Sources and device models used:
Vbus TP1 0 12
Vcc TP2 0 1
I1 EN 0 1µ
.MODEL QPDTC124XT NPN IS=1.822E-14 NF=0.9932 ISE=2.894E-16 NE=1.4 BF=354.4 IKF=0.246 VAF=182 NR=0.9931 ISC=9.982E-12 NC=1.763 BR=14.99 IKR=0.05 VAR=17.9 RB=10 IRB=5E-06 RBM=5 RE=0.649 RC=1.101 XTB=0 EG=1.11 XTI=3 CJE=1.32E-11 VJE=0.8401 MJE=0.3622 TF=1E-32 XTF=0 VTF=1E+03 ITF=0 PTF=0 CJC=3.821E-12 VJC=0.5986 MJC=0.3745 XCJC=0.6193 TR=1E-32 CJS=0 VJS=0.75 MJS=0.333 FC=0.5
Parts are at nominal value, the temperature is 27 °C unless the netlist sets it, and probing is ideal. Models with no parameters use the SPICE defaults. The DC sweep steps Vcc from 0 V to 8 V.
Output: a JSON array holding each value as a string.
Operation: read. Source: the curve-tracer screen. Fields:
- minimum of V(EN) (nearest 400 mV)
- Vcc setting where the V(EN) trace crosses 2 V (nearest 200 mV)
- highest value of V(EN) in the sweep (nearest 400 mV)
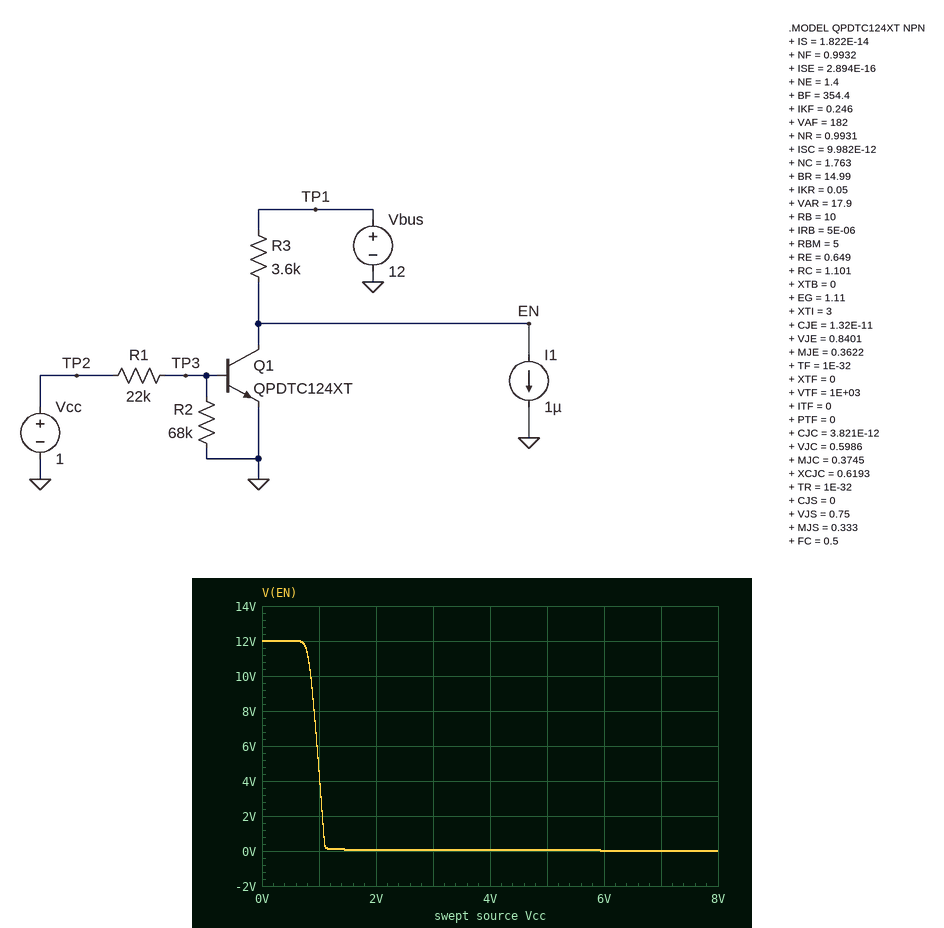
["0 V", "1.0 V", "12.0 V"]
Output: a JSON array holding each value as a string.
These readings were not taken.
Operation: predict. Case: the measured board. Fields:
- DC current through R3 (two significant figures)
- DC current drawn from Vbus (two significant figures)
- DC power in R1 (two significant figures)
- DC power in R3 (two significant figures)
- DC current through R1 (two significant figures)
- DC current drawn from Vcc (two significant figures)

["2.1 mA", "2.1 mA", "5.4 µW", "15 mW", "16 µA", "16 µA"]
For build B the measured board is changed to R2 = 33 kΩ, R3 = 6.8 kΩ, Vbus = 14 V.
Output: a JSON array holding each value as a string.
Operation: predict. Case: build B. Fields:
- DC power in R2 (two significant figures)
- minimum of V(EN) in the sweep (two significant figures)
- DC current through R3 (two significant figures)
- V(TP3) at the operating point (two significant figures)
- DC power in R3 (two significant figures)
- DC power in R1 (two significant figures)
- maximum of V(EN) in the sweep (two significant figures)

["11 µW", "17 mV", "200 µA", "590 mV", "270 µW", "7.5 µW", "14 V"]
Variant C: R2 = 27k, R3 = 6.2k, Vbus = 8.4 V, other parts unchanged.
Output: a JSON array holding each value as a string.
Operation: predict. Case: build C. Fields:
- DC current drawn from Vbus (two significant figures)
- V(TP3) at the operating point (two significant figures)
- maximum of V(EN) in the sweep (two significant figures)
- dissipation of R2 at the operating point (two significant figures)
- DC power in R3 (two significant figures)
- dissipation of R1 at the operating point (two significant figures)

["37 µA", "550 mV", "8.4 V", "11 µW", "8.6 µW", "9.2 µW"]
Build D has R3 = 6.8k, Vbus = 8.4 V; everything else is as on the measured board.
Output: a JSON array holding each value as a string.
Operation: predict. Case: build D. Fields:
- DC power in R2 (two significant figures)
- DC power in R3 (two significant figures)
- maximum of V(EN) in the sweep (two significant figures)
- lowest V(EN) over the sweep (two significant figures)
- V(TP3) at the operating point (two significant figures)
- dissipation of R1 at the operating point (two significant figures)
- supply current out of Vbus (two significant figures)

["6.1 µW", "10 mW", "8.4 V", "11 mV", "640 mV", "5.8 µW", "1.2 mA"]
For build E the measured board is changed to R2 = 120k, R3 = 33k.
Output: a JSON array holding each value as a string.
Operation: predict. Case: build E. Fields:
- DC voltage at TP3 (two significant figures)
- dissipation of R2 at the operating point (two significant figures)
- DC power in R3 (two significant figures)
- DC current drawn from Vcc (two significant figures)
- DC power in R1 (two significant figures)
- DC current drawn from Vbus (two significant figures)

["620 mV", "3.2 µW", "4.3 mW", "17 µA", "6.6 µW", "360 µA"]
